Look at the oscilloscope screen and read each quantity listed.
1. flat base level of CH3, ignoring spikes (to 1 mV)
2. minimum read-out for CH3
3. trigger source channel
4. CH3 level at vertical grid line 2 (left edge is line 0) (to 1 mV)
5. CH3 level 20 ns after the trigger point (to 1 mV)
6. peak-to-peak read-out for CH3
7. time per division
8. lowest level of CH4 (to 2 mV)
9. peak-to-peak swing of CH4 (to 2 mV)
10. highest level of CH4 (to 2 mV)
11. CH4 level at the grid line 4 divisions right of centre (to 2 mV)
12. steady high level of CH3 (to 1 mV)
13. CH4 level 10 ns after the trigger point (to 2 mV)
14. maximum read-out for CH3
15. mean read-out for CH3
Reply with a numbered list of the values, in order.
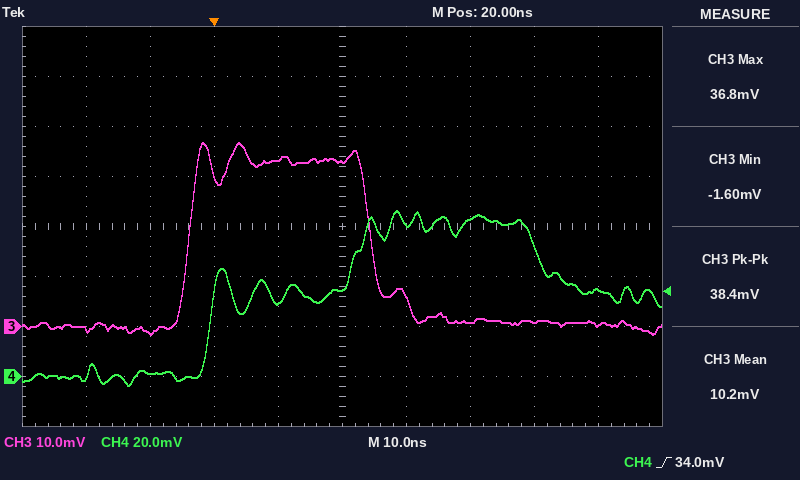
1. 1 mV
2. -1.60 mV
3. CH4
4. -1 mV
5. 33 mV
6. 38.4 mV
7. 10 ns
8. -4 mV
9. 70 mV
10. 66 mV
11. 34 mV
12. 33 mV
13. 30 mV
14. 36.8 mV
15. 10.2 mV
